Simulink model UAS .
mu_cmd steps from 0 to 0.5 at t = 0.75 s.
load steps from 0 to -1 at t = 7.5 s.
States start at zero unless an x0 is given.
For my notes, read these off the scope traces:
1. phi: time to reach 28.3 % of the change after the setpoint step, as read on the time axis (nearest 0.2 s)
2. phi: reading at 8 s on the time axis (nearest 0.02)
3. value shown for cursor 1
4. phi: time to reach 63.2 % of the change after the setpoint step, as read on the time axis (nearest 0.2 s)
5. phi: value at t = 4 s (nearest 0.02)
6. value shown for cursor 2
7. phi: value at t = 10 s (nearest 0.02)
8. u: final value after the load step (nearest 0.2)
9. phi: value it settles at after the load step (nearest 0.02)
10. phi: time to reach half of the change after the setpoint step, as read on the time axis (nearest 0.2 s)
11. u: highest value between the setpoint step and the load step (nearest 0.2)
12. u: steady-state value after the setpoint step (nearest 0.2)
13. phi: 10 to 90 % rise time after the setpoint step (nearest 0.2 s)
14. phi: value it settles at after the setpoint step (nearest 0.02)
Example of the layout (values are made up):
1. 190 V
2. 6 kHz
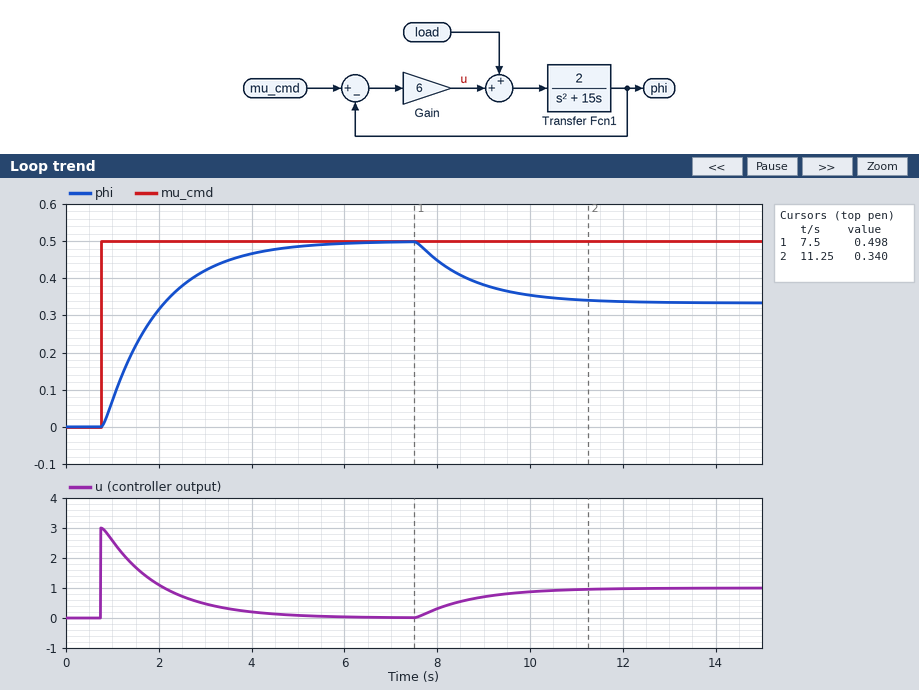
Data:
1. 1.2 s
2. 0.44
3. 0.498
4. 2.0 s
5. 0.46
6. 0.340
7. 0.36
8. 1.0
9. 0.34
10. 1.6 s
11. 3.0
12. 0.0
13. 2.6 s
14. 0.50
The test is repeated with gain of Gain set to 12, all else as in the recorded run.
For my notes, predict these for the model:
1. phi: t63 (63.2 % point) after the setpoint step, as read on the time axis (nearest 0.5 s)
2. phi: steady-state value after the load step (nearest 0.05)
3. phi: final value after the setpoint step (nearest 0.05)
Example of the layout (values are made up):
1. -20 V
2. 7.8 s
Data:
1. 1.5 s
2. 0.40
3. 0.50
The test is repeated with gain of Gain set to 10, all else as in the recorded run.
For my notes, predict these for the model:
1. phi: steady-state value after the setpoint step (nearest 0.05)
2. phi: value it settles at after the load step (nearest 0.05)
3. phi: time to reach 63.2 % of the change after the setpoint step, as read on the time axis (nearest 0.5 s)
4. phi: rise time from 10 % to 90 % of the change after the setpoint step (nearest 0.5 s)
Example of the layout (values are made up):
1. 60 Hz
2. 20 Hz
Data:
1. 0.50
2. 0.40
3. 1.5 s
4. 1.5 s
